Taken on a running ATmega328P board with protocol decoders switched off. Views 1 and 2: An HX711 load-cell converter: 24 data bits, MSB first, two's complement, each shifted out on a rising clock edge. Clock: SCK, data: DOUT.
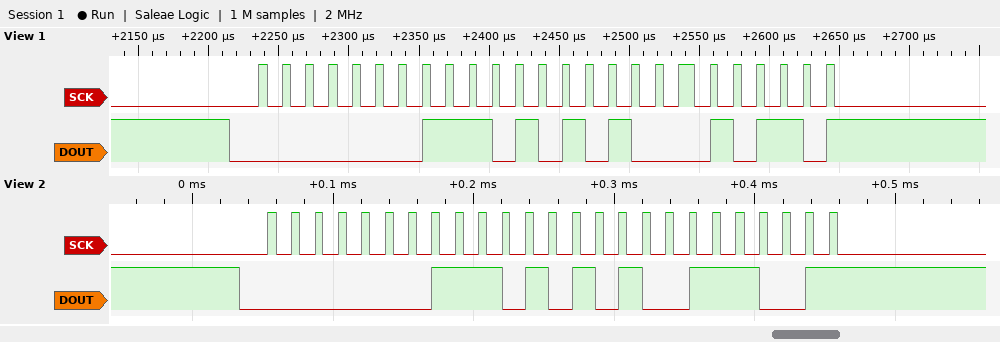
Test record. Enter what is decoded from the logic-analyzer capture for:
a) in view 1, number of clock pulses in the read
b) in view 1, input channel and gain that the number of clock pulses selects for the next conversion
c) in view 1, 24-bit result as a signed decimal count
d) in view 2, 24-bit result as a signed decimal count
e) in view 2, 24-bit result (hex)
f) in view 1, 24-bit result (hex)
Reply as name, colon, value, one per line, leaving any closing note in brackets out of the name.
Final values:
in view 1, number of clock pulses in the read: 25
in view 1, input channel and gain that the number of clock pulses selects for the next conversion: channel A, gain 128
in view 1, 24-bit result as a signed decimal count: 120086
in view 2, 24-bit result as a signed decimal count: 120121
in view 2, 24-bit result: 0x01D539
in view 1, 24-bit result: 0x01D516
